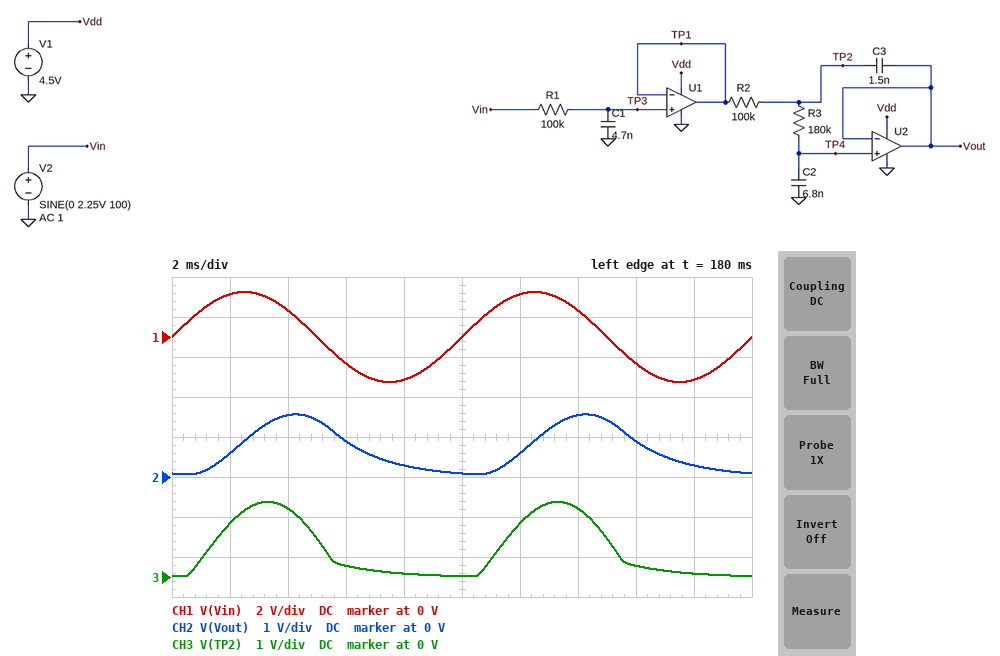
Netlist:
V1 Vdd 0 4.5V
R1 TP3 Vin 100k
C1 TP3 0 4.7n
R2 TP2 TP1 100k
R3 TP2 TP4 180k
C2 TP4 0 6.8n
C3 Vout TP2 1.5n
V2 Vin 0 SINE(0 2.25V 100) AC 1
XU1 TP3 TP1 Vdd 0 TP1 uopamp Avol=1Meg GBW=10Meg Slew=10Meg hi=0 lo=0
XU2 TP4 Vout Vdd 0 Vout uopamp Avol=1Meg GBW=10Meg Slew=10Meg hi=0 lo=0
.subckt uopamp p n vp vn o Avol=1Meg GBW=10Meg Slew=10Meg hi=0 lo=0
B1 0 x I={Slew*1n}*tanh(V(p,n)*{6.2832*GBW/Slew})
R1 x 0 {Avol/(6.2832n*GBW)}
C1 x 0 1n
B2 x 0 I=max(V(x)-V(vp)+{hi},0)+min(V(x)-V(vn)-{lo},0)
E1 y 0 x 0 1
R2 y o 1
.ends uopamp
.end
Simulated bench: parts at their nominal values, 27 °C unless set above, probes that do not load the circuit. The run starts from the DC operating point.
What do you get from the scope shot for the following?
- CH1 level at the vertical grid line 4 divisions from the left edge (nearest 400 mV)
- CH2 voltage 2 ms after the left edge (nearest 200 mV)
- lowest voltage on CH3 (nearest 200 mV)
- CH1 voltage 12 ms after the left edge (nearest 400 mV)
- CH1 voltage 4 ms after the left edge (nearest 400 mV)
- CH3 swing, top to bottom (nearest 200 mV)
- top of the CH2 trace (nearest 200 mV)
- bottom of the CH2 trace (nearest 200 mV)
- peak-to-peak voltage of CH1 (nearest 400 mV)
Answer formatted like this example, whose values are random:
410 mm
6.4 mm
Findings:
-2.0 V
600 mV
0 V
2.0 V
1.2 V
1.8 V
1.6 V
0 V
4.4 V
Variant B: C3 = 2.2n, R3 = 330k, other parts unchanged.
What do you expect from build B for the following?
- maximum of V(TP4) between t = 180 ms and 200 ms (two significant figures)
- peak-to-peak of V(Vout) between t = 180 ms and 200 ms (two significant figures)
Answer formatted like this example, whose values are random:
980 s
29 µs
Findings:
1.3 V
1.2 V
